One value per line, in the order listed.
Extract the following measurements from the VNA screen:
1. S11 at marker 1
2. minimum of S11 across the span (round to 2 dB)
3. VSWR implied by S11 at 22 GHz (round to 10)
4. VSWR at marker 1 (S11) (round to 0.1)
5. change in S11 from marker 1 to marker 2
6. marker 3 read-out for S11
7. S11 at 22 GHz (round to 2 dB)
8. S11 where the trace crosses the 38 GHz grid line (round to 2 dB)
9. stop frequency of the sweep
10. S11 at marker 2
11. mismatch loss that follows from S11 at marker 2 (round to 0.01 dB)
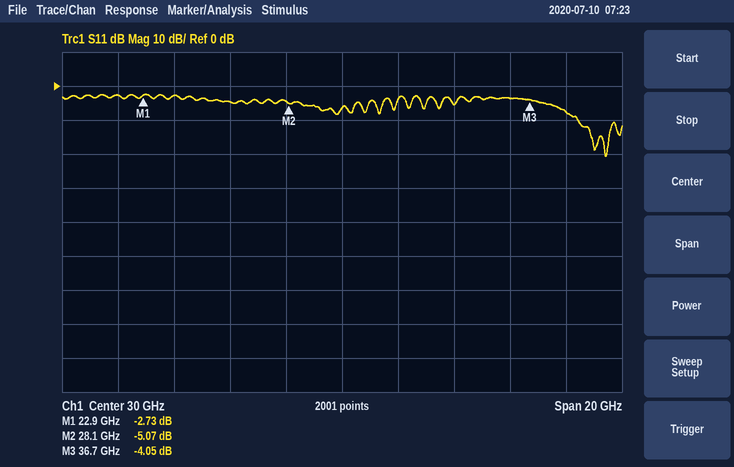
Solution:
-2.73 dB
-20 dB
10
6.4
-2.34 dB
-4.05 dB
-2 dB
-8 dB
40 GHz
-5.07 dB
1.62 dB
